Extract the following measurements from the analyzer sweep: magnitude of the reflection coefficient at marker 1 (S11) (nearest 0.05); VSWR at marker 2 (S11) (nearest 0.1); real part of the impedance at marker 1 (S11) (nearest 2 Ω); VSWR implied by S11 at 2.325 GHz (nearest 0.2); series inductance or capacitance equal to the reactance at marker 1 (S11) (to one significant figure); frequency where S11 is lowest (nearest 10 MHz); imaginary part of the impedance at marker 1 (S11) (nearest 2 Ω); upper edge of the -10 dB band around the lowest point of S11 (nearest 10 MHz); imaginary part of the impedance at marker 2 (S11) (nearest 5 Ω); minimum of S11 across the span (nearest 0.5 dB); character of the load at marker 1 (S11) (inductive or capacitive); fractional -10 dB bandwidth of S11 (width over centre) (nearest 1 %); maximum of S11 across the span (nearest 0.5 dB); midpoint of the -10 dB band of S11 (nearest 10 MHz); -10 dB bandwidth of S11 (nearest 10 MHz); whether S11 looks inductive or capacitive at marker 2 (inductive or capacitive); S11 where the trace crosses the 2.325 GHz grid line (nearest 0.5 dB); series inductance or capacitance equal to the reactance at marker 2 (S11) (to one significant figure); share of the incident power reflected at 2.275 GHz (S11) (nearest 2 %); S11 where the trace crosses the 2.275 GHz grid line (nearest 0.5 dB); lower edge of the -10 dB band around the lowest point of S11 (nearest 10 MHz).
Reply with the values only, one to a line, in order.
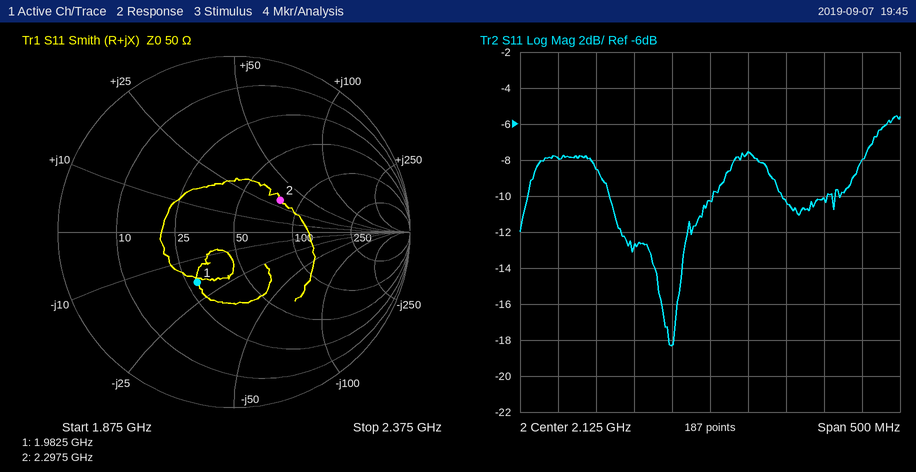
0.35
1.9
28 Ω
2.4
4 pF
2.07 GHz
-18 Ω
2.13 GHz
+30 Ω
-18.5 dB
capacitive
7 %
-5.5 dB
2.06 GHz
140 MHz
inductive
-8.0 dB
2 nH
10 %
-10.0 dB
1.99 GHz
